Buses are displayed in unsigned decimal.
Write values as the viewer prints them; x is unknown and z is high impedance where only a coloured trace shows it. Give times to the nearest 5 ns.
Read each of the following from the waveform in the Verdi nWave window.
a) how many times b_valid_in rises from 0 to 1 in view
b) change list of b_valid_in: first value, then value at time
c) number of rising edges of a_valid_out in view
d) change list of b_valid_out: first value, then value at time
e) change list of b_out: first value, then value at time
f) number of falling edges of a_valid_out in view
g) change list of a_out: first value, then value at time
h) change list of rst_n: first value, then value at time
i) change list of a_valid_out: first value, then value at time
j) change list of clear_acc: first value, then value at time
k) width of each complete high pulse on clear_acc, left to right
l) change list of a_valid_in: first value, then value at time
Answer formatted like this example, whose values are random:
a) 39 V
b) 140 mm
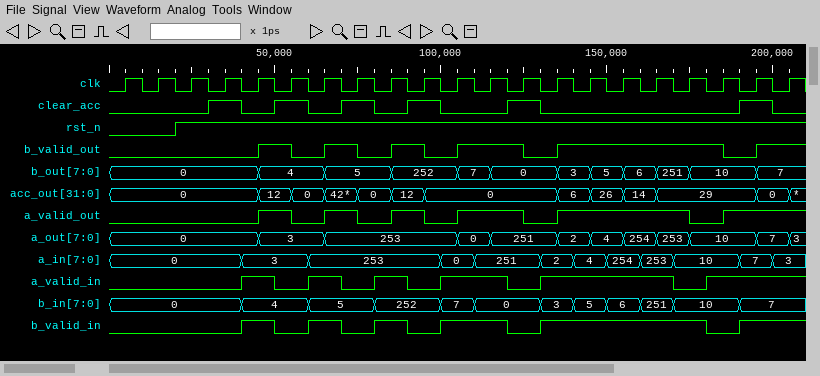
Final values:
a) 6
b) 0, 1 at 40 ns, 0 at 50 ns, 1 at 60 ns, 0 at 70 ns, 1 at 80 ns, 0 at 90 ns, 1 at 100 ns, 0 at 120 ns, 1 at 130 ns, 0 at 180 ns, 1 at 190 ns
c) 6
d) 0, 1 at 45 ns, 0 at 55 ns, 1 at 65 ns, 0 at 75 ns, 1 at 85 ns, 0 at 95 ns, 1 at 105 ns, 0 at 125 ns, 1 at 135 ns, 0 at 185 ns, 1 at 195 ns
e) 0, 4 at 45 ns, 5 at 65 ns, 252 at 85 ns, 7 at 105 ns, 0 at 115 ns, 3 at 135 ns, 5 at 145 ns, 6 at 155 ns, 251 at 165 ns, 10 at 175 ns, 7 at 195 ns
f) 5
g) 0, 3 at 45 ns, 253 at 65 ns, 0 at 105 ns, 251 at 115 ns, 2 at 135 ns, 4 at 145 ns, 254 at 155 ns, 253 at 165 ns, 10 at 175 ns, 7 at 195 ns, 3 at 205 ns
h) 0, 1 at 20 ns
i) 0, 1 at 45 ns, 0 at 55 ns, 1 at 65 ns, 0 at 75 ns, 1 at 85 ns, 0 at 95 ns, 1 at 105 ns, 0 at 125 ns, 1 at 135 ns, 0 at 175 ns, 1 at 185 ns
j) 0, 1 at 30 ns, 0 at 40 ns, 1 at 50 ns, 0 at 60 ns, 1 at 70 ns, 0 at 80 ns, 1 at 90 ns, 0 at 100 ns, 1 at 120 ns, 0 at 130 ns, 1 at 190 ns, 0 at 200 ns
k) 10 ns, 10 ns, 10 ns, 10 ns, 10 ns, 10 ns
l) 0, 1 at 40 ns, 0 at 50 ns, 1 at 60 ns, 0 at 70 ns, 1 at 80 ns, 0 at 90 ns, 1 at 100 ns, 0 at 120 ns, 1 at 130 ns, 0 at 170 ns, 1 at 180 ns
